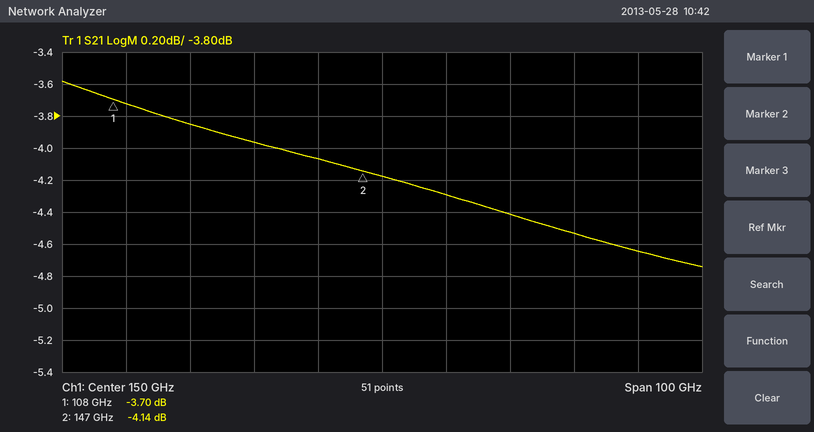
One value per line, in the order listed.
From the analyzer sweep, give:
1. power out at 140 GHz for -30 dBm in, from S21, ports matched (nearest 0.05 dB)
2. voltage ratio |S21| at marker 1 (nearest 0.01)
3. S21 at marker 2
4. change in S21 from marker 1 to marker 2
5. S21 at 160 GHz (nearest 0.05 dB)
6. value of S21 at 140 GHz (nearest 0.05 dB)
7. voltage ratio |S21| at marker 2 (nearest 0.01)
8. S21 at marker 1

-34.05 dBm
0.65
-4.14 dB
-0.44 dB
-4.30 dB
-4.05 dB
0.62
-3.70 dB
